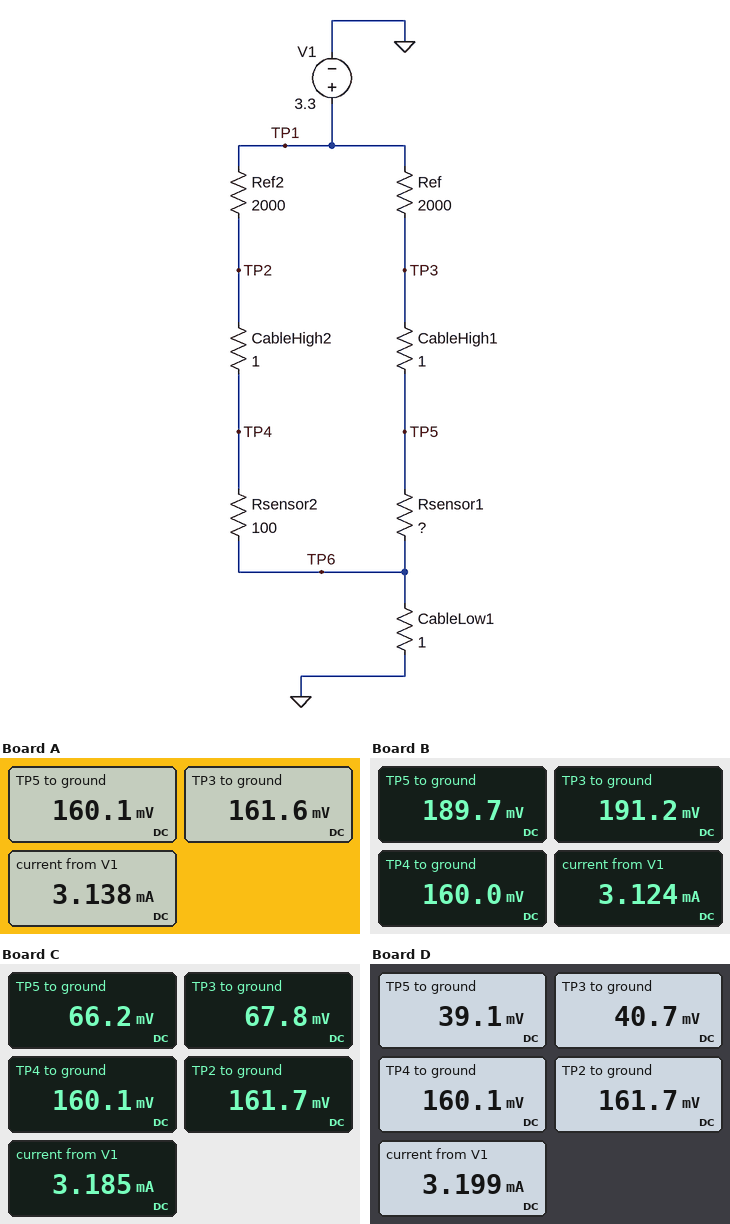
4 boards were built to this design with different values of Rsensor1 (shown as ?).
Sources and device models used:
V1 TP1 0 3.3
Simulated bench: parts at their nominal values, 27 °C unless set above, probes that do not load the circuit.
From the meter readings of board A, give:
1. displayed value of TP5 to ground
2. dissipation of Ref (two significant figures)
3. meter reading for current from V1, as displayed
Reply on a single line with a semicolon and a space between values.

160.1 mV; 4.9 mW; 3.138 mA
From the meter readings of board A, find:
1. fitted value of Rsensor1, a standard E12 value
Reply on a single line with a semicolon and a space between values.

100 Ω
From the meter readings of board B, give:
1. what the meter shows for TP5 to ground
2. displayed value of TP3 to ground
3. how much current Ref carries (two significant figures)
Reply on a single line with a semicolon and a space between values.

189.7 mV; 191.2 mV; 1.6 mA
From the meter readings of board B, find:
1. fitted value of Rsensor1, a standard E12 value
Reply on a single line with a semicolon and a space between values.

120 Ω
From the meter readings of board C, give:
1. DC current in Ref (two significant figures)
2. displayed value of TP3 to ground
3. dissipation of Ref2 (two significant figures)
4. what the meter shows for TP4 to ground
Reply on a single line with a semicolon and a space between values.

1.6 mA; 67.8 mV; 4.9 mW; 160.1 mV
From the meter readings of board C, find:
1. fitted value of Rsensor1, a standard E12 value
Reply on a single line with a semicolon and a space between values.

39 Ω
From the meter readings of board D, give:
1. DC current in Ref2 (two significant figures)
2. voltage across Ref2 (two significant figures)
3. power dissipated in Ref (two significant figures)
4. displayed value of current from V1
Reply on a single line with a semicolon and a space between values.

1.6 mA; 3.1 V; 5.3 mW; 3.199 mA
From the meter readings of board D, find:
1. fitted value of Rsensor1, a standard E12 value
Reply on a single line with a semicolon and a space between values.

22 Ω
